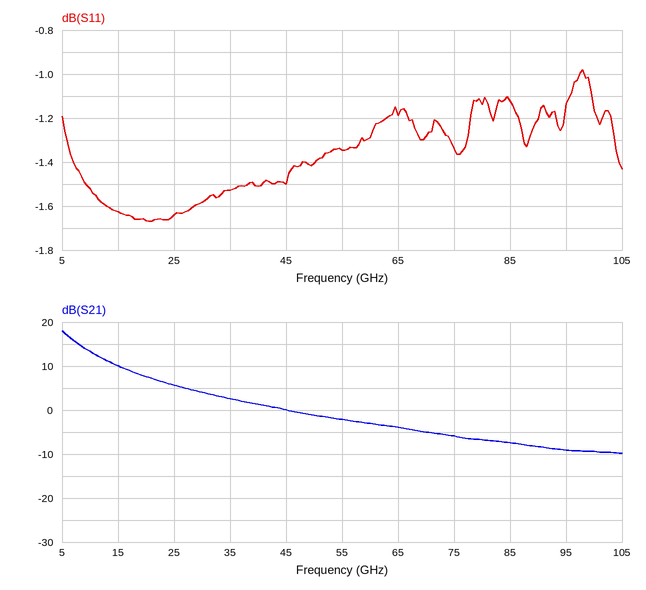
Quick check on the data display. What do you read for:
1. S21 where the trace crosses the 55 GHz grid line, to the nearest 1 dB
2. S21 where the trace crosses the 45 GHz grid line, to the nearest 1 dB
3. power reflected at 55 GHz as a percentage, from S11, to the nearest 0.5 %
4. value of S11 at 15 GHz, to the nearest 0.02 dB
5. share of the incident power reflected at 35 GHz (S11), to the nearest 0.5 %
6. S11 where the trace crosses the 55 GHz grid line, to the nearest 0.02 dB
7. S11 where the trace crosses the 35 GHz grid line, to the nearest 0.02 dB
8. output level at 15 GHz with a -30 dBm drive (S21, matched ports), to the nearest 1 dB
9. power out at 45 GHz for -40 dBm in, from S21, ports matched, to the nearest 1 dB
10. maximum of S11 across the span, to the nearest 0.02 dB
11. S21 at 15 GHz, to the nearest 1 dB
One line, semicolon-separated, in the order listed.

-2 dB; 0 dB; 73.5 %; -1.62 dB; 70.5 %; -1.34 dB; -1.52 dB; -20 dBm; -40 dBm; -0.98 dB; 10 dB
